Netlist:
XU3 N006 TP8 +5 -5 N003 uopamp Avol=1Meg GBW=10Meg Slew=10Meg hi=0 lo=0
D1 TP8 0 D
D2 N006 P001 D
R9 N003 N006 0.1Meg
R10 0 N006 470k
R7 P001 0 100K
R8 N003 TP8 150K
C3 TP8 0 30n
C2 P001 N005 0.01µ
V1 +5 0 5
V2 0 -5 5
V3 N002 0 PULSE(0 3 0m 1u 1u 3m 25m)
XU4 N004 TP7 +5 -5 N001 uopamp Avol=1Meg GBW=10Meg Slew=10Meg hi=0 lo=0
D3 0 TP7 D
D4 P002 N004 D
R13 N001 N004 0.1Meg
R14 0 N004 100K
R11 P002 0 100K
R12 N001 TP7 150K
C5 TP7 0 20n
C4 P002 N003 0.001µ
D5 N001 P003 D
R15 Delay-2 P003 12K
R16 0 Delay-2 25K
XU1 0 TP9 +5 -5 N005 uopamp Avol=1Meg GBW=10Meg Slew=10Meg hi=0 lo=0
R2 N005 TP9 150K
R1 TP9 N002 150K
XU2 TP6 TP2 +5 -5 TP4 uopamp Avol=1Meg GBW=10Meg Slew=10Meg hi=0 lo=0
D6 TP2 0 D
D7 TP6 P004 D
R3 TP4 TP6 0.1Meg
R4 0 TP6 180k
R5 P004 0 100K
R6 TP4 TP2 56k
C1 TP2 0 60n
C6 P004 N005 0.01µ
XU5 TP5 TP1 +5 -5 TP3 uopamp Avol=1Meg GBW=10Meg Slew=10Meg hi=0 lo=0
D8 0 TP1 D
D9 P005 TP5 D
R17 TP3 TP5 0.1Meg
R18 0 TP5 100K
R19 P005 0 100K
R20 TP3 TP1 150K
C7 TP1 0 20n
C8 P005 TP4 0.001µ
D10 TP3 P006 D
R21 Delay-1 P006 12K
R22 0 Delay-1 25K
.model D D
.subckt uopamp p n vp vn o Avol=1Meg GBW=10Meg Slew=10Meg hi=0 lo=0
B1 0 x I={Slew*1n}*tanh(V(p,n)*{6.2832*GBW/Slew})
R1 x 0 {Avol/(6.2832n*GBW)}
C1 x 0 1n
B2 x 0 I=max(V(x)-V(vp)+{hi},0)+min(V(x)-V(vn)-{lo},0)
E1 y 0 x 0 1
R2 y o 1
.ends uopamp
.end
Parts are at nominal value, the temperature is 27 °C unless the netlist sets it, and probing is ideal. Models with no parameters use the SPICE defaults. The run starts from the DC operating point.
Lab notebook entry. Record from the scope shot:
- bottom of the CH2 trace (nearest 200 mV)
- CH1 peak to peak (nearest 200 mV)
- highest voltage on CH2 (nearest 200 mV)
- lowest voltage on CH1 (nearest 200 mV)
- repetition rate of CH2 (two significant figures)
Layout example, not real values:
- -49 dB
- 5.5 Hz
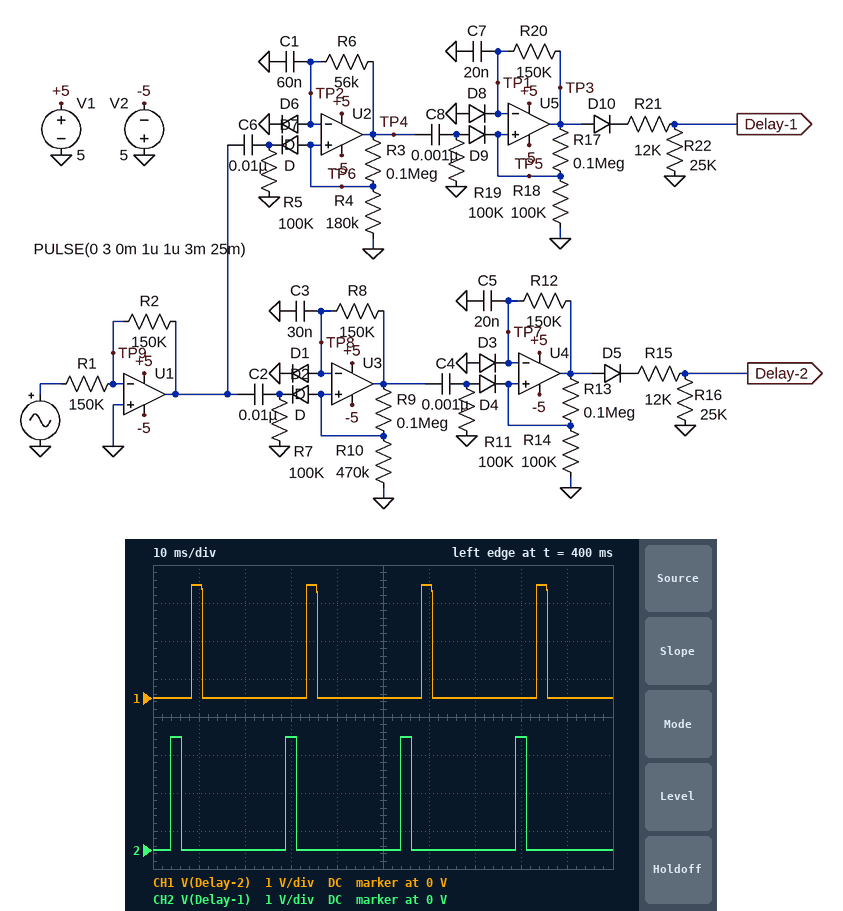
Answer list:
- 0 V
- 3.0 V
- 3.0 V
- 0 V
- 40 Hz
